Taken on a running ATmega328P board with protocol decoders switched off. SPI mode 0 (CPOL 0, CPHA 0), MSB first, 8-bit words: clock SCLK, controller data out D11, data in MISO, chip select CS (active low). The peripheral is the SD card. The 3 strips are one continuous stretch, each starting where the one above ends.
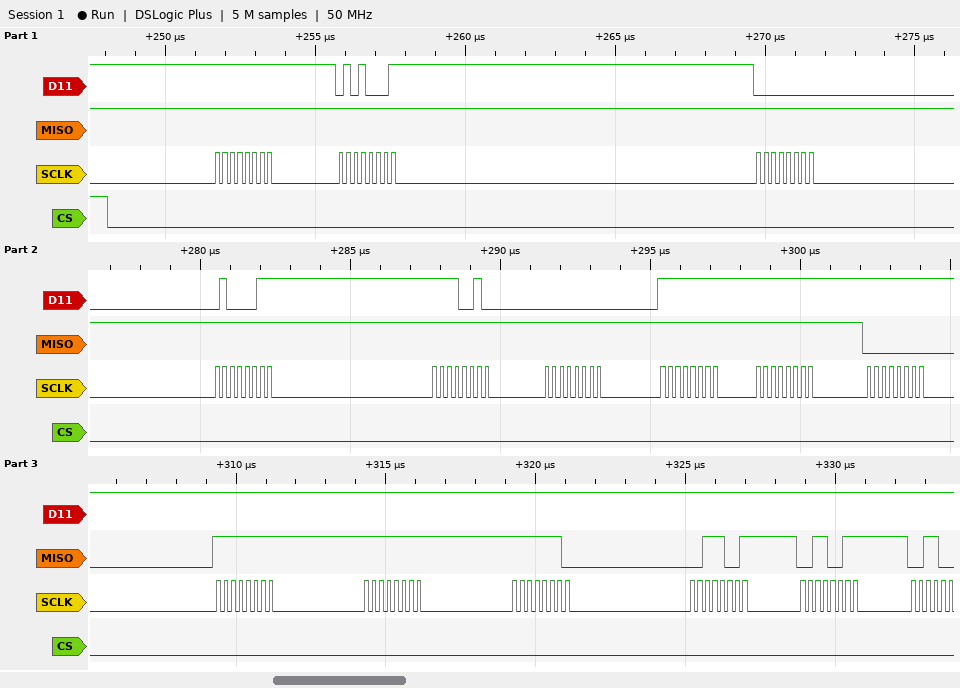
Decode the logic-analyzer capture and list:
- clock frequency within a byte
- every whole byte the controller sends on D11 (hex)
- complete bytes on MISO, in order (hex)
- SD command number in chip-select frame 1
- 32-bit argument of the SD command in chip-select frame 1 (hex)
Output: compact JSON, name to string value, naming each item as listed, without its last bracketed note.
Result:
{"clock frequency within a byte": "4 MHz", "every whole byte the controller sends on D11": "FF 51 00 43 F2 00 FF FF FF FF FF FF FF FF", "complete bytes on MISO, in order": "FF FF FF FF FF FF FF FF 00 FF FF FE 39 33", "SD command number in chip-select frame 1": "CMD17", "32-bit argument of the SD command in chip-select frame 1": "0x0043F200"}
